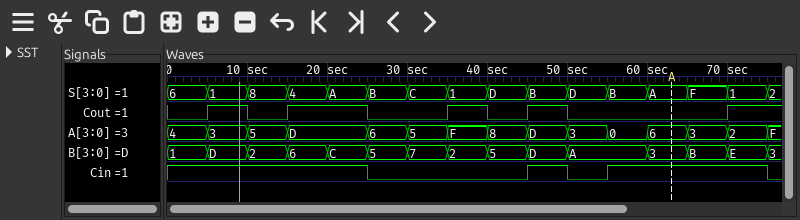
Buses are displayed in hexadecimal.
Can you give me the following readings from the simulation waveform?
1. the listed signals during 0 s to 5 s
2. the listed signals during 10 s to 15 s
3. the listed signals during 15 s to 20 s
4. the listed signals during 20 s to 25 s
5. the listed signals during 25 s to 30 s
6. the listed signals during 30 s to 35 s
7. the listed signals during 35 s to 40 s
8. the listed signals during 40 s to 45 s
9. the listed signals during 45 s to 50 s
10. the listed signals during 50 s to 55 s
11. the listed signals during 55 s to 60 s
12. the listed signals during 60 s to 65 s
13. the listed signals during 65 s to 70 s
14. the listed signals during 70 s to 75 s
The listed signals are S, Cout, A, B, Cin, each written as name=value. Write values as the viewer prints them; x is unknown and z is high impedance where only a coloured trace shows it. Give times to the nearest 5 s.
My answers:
S=6, Cout=0, A=4, B=1, Cin=1
S=8, Cout=0, A=5, B=2, Cin=1
S=4, Cout=1, A=D, B=6, Cin=1
S=A, Cout=1, A=D, B=C, Cin=1
S=B, Cout=0, A=6, B=5, Cin=0
S=C, Cout=0, A=5, B=7, Cin=0
S=1, Cout=1, A=F, B=2, Cin=0
S=D, Cout=0, A=8, B=5, Cin=0
S=B, Cout=1, A=D, B=D, Cin=1
S=D, Cout=0, A=3, B=A, Cin=0
S=B, Cout=0, A=0, B=A, Cin=1
S=A, Cout=0, A=6, B=3, Cin=1
S=F, Cout=0, A=3, B=B, Cin=1
S=1, Cout=1, A=2, B=E, Cin=1
